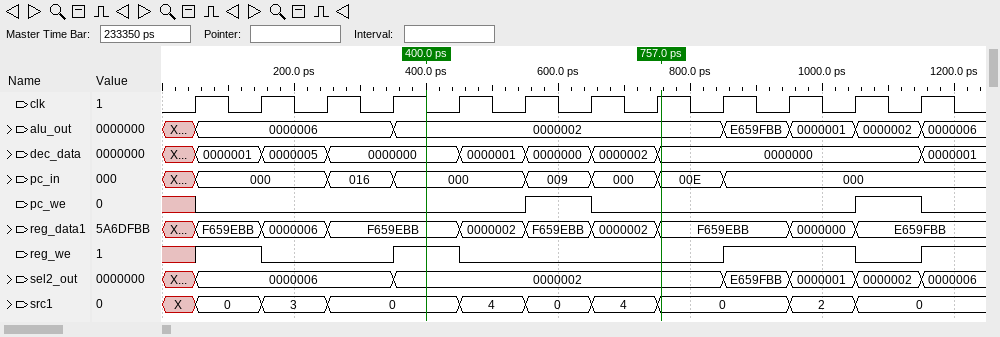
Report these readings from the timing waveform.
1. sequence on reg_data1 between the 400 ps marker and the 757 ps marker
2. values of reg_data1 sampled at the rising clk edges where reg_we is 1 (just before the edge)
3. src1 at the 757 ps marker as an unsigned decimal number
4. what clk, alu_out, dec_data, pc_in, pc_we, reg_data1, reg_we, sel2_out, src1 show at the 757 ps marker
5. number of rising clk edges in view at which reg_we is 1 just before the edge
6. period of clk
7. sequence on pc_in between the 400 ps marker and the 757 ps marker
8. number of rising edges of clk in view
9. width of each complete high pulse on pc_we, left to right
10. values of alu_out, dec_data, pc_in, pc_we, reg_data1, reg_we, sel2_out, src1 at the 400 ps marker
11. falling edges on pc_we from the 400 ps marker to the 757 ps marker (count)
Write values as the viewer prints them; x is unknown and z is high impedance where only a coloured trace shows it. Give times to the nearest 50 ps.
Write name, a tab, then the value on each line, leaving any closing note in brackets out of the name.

sequence on reg_data1 between the 400 ps marker and the 757 ps marker	F659EBB, 0000002, F659EBB, 0000002, F659EBB
values of reg_data1 sampled at the rising clk edges where reg_we is 1	F659EBB, F659EBB, F659EBB, 0000000
src1 at the 757 ps marker as an unsigned decimal number	0
what clk, alu_out, dec_data, pc_in, pc_we, reg_data1, reg_we, sel2_out, src1 show at the 757 ps marker	clk=1, alu_out=0000002, dec_data=0000000, pc_in=00E, pc_we=0, reg_data1=F659EBB, reg_we=0, sel2_out=0000002, src1=0
number of rising clk edges in view at which reg_we is 1 just before the edge	4
period of clk	100 ps
sequence on pc_in between the 400 ps marker and the 757 ps marker	000, 009, 000, 00E
number of rising edges of clk in view	12
width of each complete high pulse on pc_we, left to right	100 ps, 100 ps
values of alu_out, dec_data, pc_in, pc_we, reg_data1, reg_we, sel2_out, src1 at the 400 ps marker	alu_out=0000002, dec_data=0000000, pc_in=000, pc_we=0, reg_data1=F659EBB, reg_we=1, sel2_out=0000002, src1=0
falling edges on pc_we from the 400 ps marker to the 757 ps marker	1
